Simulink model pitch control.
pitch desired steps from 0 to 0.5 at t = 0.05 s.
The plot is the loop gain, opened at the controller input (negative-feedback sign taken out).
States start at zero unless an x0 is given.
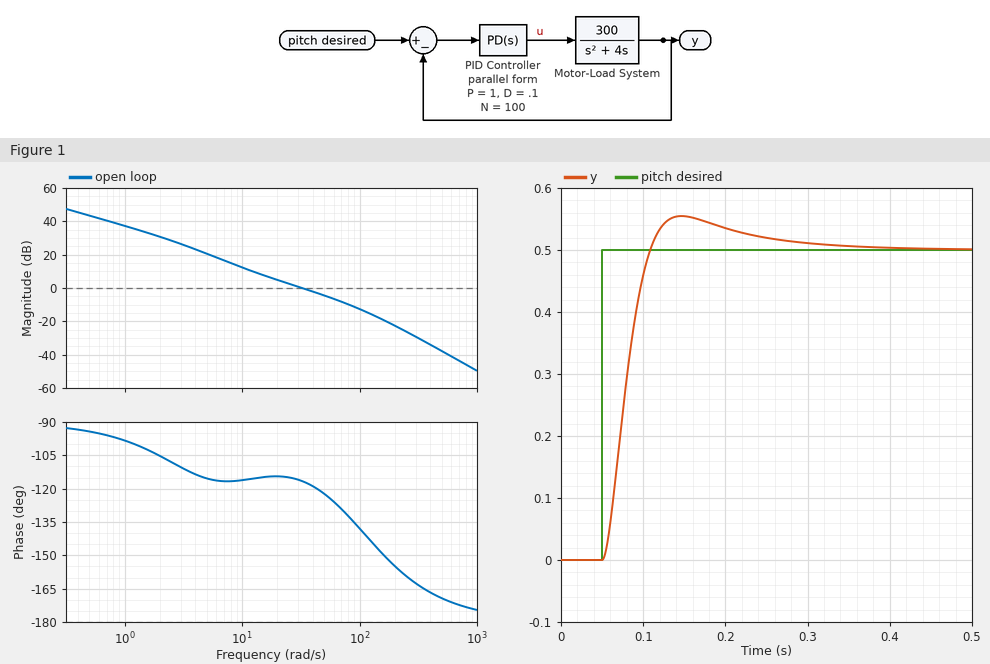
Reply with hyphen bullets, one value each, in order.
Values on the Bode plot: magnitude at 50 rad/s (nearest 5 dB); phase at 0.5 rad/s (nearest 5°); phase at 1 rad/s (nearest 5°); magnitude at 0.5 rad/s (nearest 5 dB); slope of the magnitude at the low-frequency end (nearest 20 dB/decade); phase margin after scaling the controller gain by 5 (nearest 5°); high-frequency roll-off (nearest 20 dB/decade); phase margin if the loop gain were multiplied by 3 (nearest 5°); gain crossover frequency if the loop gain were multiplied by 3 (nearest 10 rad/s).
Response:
- -5 dB
- -95°
- -100°
- 45 dB
- -20 dB/decade
- 40°
- -40 dB/decade
- 50°
- 80 rad/s
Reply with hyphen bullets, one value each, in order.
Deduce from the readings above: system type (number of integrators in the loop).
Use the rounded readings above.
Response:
- 1
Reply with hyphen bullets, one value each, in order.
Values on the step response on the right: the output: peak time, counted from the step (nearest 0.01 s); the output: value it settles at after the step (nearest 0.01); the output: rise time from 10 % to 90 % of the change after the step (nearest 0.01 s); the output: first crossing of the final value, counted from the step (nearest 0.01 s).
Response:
- 0.10 s
- 0.50
- 0.04 s
- 0.06 s
